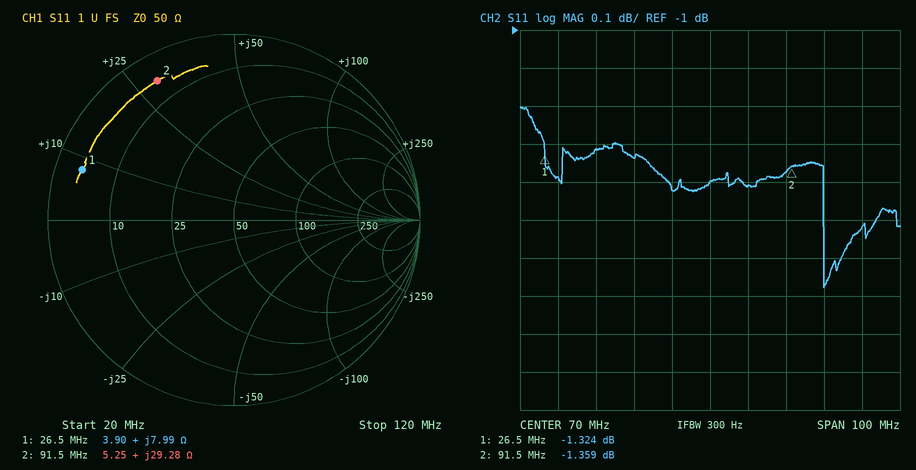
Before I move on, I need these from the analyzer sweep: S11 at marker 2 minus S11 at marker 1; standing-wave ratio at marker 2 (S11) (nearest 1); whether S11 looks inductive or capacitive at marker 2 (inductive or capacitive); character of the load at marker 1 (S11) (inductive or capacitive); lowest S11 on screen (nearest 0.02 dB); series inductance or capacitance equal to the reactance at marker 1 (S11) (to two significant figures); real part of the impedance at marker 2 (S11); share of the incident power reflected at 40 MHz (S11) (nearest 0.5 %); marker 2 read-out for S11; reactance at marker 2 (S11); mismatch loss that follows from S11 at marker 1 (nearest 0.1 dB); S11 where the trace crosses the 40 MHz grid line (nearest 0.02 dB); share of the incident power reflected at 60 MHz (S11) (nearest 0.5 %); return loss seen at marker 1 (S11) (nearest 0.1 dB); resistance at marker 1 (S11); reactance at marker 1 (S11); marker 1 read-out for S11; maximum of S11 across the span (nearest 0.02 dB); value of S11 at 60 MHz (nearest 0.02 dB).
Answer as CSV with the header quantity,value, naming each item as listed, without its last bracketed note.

quantity,value
S11 at marker 2 minus S11 at marker 1,-0.035 dB
standing-wave ratio at marker 2 (S11),13
whether S11 looks inductive or capacitive at marker 2,inductive
character of the load at marker 1 (S11),inductive
lowest S11 on screen,-1.68 dB
series inductance or capacitance equal to the reactance at marker 1 (S11),48 nH
real part of the impedance at marker 2,5.25 Ω
share of the incident power reflected at 40 MHz (S11),74.0 %
marker 2 read-out for S11,-1.359 dB
reactance at marker 2,+29.28 Ω
mismatch loss that follows from S11 at marker 1,5.8 dB
S11 where the trace crosses the 40 MHz grid line,-1.32 dB
share of the incident power reflected at 60 MHz (S11),72.0 %
return loss seen at marker 1 (S11),1.3 dB
resistance at marker 1,3.90 Ω
reactance at marker 1,+7.99 Ω
marker 1 read-out for S11,-1.324 dB
maximum of S11 across the span,-1.20 dB
value of S11 at 60 MHz,-1.42 dB
